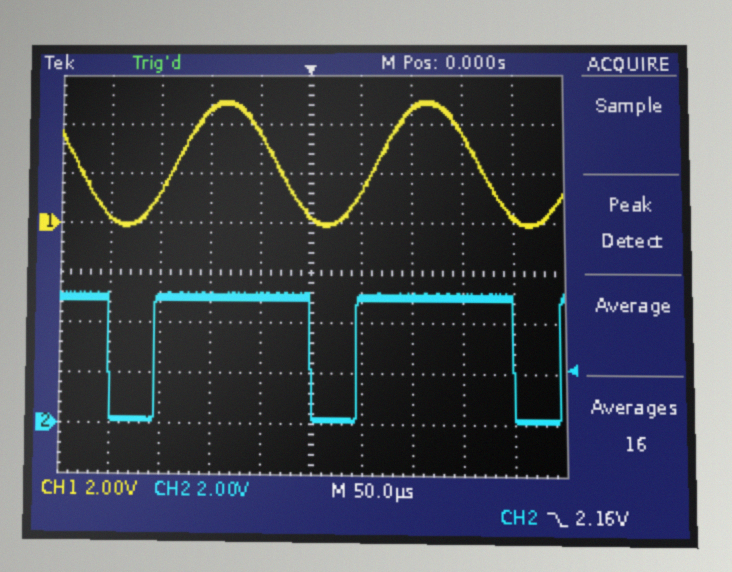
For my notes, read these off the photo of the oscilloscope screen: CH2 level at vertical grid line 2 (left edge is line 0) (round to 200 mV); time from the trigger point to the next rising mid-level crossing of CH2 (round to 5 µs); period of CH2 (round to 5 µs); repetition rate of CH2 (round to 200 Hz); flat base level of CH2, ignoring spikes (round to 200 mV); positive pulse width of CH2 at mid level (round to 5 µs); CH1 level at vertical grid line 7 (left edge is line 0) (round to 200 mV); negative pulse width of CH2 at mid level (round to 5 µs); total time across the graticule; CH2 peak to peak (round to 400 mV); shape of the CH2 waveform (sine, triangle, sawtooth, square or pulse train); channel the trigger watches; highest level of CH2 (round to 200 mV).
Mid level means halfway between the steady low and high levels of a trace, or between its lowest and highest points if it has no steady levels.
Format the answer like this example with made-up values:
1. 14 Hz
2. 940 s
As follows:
1. 5.0 V
2. 45 µs
3. 200 µs
4. 5.0 kHz
5. 200 mV
6. 155 µs
7. 4.6 V
8. 45 µs
9. 500 µs
10. 5.2 V
11. pulse train
12. CH2
13. 5.2 V
